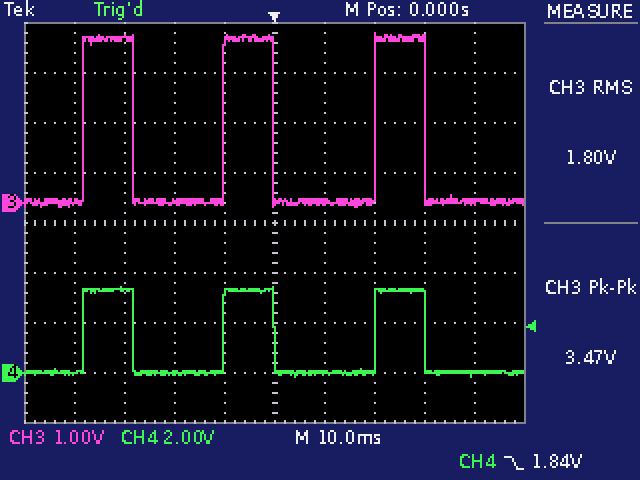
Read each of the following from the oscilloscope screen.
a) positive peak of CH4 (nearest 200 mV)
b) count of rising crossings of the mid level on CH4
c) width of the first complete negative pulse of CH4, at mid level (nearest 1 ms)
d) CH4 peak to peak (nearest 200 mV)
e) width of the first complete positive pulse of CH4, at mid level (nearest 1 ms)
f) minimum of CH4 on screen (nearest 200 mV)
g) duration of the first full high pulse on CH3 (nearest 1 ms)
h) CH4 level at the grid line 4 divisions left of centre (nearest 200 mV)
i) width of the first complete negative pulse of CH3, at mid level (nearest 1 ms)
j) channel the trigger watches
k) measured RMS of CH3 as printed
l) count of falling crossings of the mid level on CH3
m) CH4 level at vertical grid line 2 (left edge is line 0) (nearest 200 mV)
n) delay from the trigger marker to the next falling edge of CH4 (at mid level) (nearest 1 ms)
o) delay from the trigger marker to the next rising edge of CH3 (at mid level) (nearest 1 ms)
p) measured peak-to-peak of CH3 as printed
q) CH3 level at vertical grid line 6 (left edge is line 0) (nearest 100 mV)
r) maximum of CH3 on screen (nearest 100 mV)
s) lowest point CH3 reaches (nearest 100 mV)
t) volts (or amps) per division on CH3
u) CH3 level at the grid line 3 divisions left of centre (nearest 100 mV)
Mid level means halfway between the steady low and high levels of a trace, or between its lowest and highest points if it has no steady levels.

3.4 V
3
18 ms
3.6 V
10 ms
-200 mV
10 ms
0.0 V
18 ms
CH4
1.80 V
3
3.4 V
30 ms
20 ms
3.47 V
0.0 V
3.4 V
-100 mV
1 V
3.3 V
